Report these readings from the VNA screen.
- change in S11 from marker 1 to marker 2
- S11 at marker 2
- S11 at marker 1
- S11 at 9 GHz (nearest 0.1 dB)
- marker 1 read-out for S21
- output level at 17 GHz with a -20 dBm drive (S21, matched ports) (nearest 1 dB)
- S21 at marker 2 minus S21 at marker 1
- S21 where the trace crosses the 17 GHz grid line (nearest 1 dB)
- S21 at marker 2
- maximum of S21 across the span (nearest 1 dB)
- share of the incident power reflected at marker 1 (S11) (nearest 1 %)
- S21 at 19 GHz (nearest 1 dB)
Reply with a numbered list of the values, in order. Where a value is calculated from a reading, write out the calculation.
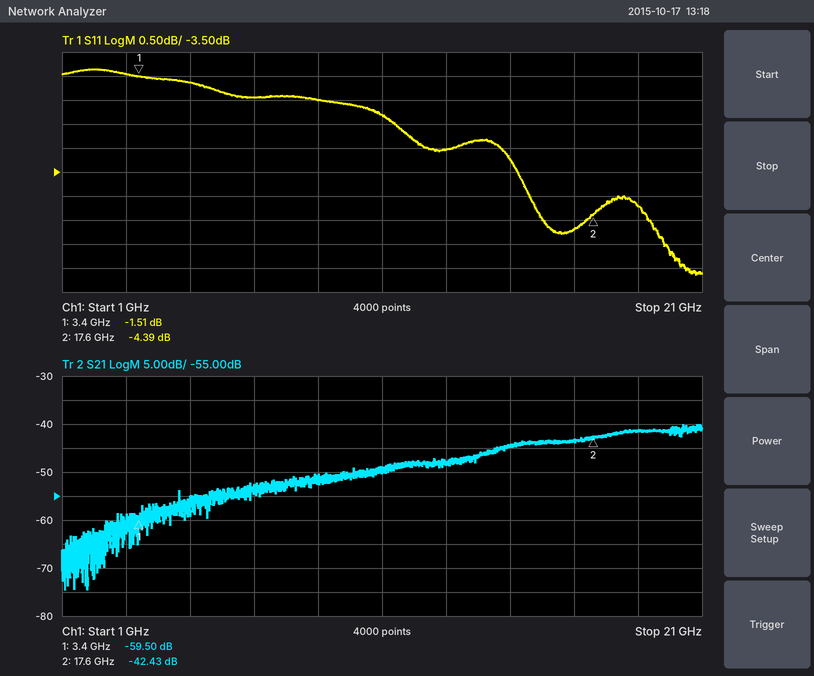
1. -4.39 − (-1.51) = -2.88 dB
2. -4.39 dB
3. -1.51 dB
4. -2.0 dB
5. -59.50 dB
6. -20 dBm + (-43 dB) = -63 dBm
7. -42.43 − (-59.5) = 17.07 dB
8. -43 dB
9. -42.43 dB
10. -40 dB
11. 10^(-1.51/10) ≈ 71 %
12. -41 dB
